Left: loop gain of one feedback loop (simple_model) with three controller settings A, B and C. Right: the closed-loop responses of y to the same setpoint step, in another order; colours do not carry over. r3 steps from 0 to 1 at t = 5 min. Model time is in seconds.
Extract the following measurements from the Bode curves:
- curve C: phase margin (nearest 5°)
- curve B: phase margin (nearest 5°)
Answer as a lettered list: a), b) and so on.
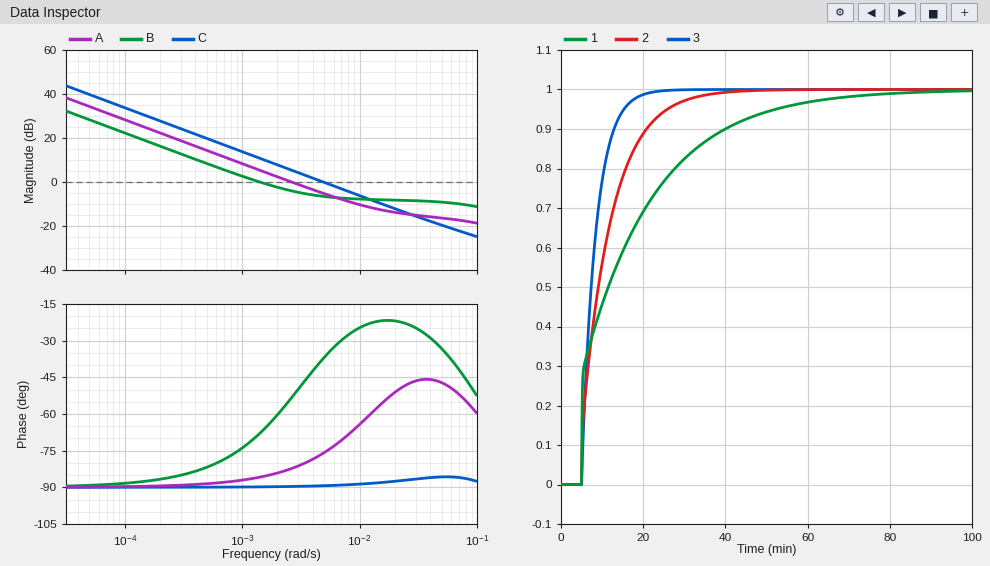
a) 90°
b) 110°
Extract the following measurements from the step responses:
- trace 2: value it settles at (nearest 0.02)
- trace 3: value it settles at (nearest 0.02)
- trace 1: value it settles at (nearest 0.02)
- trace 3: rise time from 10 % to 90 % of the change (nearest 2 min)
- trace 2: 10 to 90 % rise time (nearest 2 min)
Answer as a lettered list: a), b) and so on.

a) 1.00
b) 1.00
c) 1.00
d) 8 min
e) 16 min
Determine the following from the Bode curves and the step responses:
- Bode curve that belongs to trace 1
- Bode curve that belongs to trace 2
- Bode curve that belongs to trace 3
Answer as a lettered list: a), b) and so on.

a) B
b) A
c) C
